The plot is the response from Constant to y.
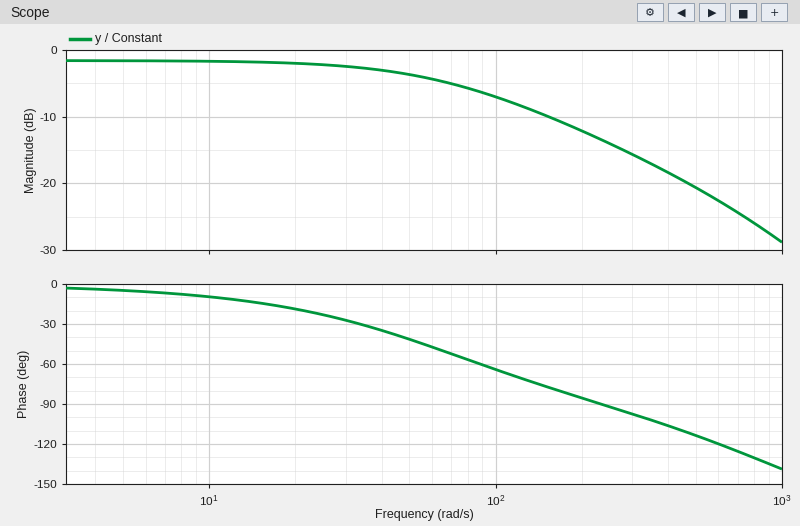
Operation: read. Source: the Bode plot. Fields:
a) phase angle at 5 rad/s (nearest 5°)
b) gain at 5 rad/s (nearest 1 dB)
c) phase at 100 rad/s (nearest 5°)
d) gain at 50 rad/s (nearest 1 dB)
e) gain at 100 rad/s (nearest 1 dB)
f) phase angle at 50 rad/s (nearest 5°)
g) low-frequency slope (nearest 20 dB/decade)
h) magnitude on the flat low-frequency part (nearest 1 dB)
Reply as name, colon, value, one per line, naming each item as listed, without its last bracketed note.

phase angle at 5 rad/s: -5°
gain at 5 rad/s: -2 dB
phase at 100 rad/s: -65°
gain at 50 rad/s: -4 dB
gain at 100 rad/s: -7 dB
phase angle at 50 rad/s: -40°
low-frequency slope: 0 dB/decade
magnitude on the flat low-frequency part: -2 dB
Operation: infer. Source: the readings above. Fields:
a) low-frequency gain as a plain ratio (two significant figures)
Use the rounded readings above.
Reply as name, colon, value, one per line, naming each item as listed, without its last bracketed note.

low-frequency gain as a plain ratio: 0.79
